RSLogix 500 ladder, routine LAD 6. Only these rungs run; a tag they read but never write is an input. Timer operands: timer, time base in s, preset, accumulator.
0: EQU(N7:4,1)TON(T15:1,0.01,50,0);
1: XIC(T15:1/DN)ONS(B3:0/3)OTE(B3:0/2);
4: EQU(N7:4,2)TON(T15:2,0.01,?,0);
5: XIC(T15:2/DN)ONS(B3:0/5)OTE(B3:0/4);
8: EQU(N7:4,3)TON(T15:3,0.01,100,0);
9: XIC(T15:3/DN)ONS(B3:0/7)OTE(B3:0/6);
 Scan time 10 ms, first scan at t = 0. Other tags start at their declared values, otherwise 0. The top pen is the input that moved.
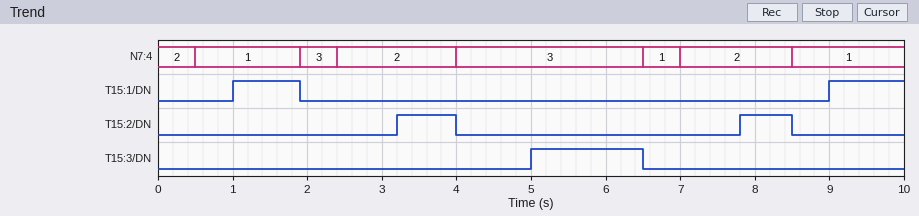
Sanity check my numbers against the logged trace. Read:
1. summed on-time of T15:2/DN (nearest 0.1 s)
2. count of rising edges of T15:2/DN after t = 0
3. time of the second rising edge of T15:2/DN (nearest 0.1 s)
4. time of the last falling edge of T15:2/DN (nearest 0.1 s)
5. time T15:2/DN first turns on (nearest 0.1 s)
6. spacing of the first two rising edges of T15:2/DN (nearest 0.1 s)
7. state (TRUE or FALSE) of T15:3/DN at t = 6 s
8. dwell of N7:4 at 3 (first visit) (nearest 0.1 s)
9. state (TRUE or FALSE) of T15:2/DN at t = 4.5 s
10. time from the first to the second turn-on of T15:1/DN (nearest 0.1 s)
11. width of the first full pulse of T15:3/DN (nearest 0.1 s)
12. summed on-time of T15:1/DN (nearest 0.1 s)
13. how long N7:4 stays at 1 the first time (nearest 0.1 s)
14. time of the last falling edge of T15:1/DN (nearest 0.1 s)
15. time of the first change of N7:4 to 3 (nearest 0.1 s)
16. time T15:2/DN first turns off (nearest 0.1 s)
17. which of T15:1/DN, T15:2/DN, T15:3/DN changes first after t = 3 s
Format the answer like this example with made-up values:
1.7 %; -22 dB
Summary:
1.5 s; 2; 7.8 s; 8.5 s; 3.2 s; 4.6 s; TRUE; 0.5 s; FALSE; 8.0 s; 1.5 s; 1.9 s; 1.4 s; 1.9 s; 1.9 s; 4.0 s; T15:2/DN
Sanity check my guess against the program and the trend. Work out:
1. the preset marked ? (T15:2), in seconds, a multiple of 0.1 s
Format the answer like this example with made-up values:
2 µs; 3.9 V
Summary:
0.8 s
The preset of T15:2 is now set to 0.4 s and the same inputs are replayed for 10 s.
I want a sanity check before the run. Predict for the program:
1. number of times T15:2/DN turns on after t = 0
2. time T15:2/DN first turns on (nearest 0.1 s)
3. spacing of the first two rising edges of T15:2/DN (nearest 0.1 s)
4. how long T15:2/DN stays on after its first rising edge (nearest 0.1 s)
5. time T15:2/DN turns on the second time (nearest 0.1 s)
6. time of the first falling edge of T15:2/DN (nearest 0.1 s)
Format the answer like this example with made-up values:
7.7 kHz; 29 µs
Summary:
3; 0.4 s; 2.4 s; 0.1 s; 2.8 s; 0.5 s
